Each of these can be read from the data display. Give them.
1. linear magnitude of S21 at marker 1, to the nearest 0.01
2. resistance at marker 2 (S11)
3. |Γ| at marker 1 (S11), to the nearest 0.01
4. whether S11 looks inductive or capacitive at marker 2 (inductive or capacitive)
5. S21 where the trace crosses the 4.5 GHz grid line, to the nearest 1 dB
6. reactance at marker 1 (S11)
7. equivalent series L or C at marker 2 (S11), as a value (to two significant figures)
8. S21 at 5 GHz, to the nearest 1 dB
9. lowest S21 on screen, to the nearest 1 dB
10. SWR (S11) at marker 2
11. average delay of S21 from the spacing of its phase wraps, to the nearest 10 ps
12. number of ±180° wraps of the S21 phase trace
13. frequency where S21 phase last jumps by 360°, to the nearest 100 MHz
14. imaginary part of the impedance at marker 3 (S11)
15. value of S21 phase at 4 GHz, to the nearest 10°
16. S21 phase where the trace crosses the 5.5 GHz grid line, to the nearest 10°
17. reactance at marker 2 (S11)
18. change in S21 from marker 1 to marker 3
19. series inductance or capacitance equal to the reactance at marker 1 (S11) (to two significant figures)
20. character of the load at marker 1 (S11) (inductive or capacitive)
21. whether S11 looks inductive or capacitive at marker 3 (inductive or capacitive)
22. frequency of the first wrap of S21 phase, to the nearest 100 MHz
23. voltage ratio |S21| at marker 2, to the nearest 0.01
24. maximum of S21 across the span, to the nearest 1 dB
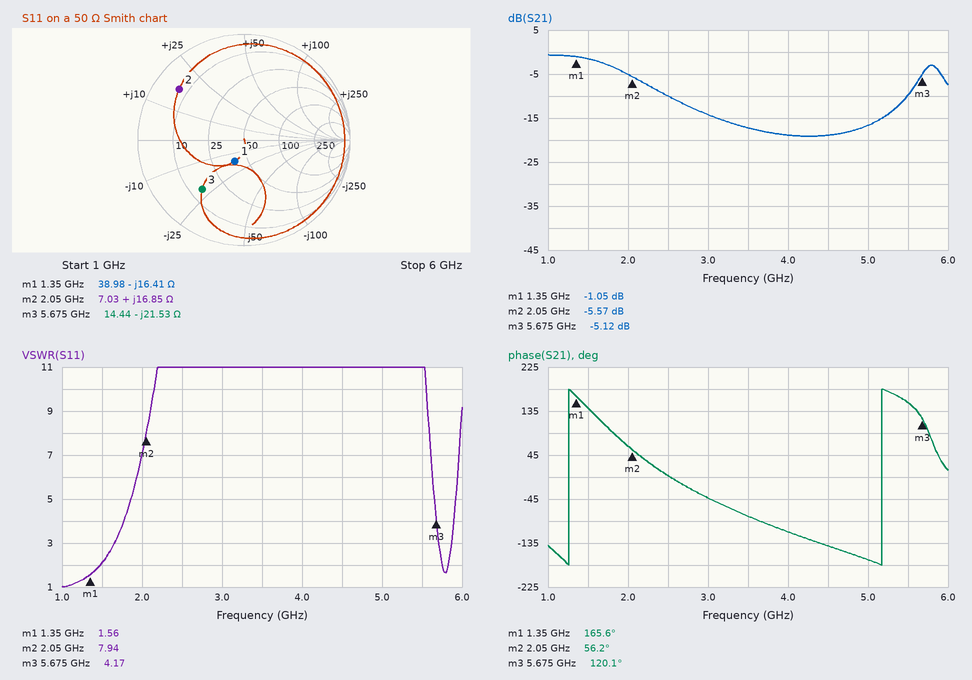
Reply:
0.89
7.03 Ω
0.22
inductive
-19 dB
-16.41 Ω
1.3 nH
-17 dB
-19 dB
7.94
260 ps
2
5.2 GHz
-21.53 Ω
-110°
150°
+16.85 Ω
-4.07 dB
7.2 pF
capacitive
capacitive
1.3 GHz
0.53
-1 dB
